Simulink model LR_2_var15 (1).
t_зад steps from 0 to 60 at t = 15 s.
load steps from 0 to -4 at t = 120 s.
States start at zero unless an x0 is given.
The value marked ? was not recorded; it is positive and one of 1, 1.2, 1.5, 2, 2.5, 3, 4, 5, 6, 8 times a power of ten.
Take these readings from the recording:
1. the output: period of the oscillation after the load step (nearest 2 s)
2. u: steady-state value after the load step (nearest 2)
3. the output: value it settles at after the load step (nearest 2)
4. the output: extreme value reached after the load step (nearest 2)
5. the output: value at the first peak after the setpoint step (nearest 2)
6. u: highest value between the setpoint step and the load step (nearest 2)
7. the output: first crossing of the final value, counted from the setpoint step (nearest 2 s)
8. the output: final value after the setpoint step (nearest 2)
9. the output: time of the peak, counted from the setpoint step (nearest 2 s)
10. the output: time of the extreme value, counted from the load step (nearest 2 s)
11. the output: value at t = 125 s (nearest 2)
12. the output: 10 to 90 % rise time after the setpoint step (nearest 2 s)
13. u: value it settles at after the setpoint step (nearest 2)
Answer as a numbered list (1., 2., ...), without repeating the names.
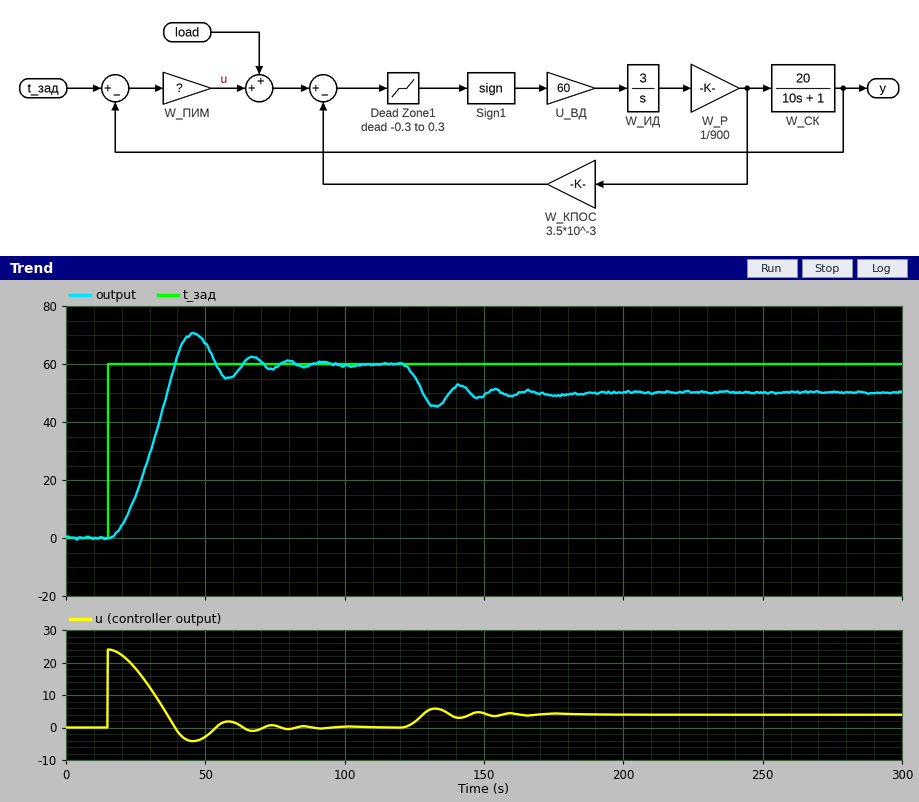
1. 16 s
2. 4
3. 50
4. 46
5. 70
6. 24
7. 24 s
8. 60
9. 30 s
10. 12 s
11. 56
12. 16 s
13. 0
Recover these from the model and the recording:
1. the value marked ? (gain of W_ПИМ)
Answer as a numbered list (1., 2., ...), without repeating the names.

1. 0.4
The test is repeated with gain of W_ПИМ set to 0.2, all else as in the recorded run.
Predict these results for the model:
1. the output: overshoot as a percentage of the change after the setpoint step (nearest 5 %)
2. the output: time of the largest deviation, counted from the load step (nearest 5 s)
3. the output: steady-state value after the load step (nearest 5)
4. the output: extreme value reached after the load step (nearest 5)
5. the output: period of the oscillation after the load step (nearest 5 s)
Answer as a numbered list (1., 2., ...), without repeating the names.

1. 20 %
2. 15 s
3. 40
4. 35
5. 20 s
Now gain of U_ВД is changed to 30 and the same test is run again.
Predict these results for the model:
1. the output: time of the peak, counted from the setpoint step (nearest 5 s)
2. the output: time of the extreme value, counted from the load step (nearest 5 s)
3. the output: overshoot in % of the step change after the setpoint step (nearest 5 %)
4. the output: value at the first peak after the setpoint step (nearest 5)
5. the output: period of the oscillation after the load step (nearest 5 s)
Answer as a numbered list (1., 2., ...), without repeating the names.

1. 45 s
2. 15 s
3. 10 %
4. 65
5. 20 s
